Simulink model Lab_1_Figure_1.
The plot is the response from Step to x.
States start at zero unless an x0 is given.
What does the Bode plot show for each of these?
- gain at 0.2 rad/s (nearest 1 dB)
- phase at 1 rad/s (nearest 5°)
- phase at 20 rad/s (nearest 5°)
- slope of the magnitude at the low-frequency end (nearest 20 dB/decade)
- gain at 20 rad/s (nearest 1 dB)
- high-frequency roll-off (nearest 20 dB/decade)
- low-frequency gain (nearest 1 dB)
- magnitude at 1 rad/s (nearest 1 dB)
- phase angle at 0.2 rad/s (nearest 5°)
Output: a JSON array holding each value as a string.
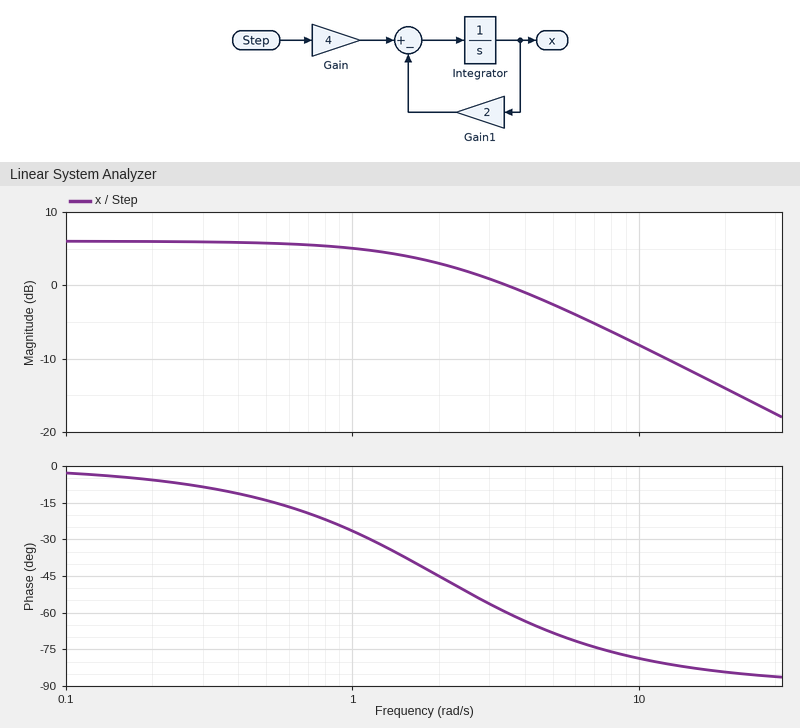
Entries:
["6 dB", "-25°", "-85°", "0 dB/decade", "-14 dB", "-20 dB/decade", "6 dB", "5 dB", "-5°"]
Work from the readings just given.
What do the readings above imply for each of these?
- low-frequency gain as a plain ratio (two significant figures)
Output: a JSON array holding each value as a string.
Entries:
["2.0"]
